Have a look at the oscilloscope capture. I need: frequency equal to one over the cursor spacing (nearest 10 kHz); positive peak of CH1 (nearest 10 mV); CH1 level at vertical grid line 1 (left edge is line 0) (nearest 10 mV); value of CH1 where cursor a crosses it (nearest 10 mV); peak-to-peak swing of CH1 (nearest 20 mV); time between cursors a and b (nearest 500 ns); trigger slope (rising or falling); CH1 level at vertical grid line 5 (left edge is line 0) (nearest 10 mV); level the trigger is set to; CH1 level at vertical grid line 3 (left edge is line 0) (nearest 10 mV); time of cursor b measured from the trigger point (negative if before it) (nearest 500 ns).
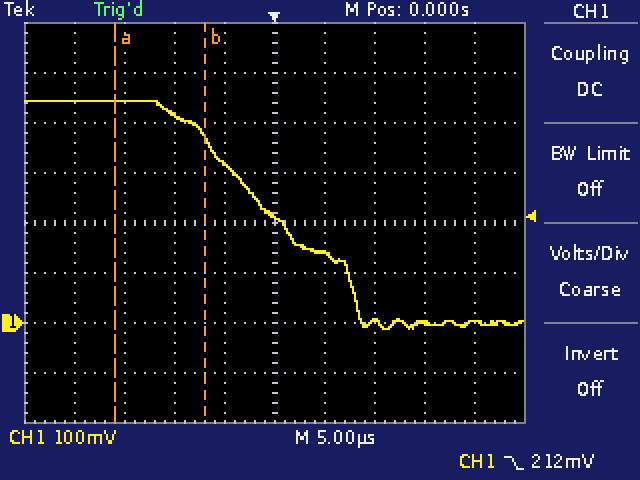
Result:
110 kHz
440 mV
440 mV
440 mV
460 mV
9.0 µs
falling
210 mV
212 mV
420 mV
-7.0 µs
